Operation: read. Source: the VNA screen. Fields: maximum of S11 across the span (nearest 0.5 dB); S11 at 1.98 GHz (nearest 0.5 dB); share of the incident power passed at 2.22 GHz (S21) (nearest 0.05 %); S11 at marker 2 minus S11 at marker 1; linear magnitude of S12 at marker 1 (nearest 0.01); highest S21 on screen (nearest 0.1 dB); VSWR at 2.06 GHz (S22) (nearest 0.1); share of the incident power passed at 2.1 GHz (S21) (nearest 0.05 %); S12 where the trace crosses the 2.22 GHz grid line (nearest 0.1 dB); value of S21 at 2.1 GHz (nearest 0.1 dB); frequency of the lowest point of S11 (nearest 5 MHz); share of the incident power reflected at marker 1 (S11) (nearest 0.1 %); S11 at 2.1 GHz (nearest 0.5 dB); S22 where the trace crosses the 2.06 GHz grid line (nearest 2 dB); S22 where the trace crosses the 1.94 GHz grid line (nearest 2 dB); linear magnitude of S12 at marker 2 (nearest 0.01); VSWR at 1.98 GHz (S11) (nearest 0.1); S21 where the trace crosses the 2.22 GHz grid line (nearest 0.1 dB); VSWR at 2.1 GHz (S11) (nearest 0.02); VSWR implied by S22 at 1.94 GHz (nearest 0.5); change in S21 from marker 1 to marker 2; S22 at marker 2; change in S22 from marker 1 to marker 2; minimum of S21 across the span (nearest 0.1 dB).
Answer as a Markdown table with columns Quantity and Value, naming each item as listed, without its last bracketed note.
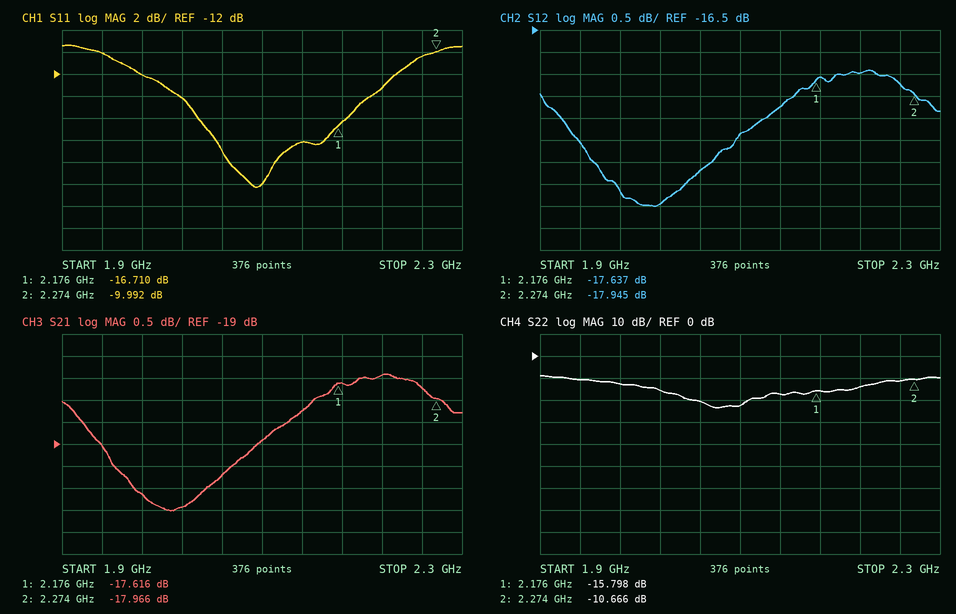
| Quantity | Value |
|---|---|
| maximum of S11 across the span | -9.5 dB |
| S11 at 1.98 GHz | -12.0 dB |
| share of the incident power passed at 2.22 GHz (S21) | 1.80 % |
| S11 at marker 2 minus S11 at marker 1 | 6.718 dB |
| linear magnitude of S12 at marker 1 | 0.13 |
| highest S21 on screen | -17.4 dB |
| VSWR at 2.06 GHz (S22) | 1.2 |
| share of the incident power passed at 2.1 GHz (S21) | 1.30 % |
| S12 where the trace crosses the 2.22 GHz grid line | -17.5 dB |
| value of S21 at 2.1 GHz | -18.9 dB |
| frequency of the lowest point of S11 | 2.095 GHz |
| share of the incident power reflected at marker 1 (S11) | 2.1 % |
| S11 at 2.1 GHz | -22.0 dB |
| S22 where the trace crosses the 2.06 GHz grid line | -20 dB |
| S22 where the trace crosses the 1.94 GHz grid line | -10 dB |
| linear magnitude of S12 at marker 2 | 0.13 |
| VSWR at 1.98 GHz (S11) | 1.7 |
| S21 where the trace crosses the 2.22 GHz grid line | -17.4 dB |
| VSWR at 2.1 GHz (S11) | 1.18 |
| VSWR implied by S22 at 1.94 GHz | 2.0 |
| change in S21 from marker 1 to marker 2 | -0.350 dB |
| S22 at marker 2 | -10.666 dB |
| change in S22 from marker 1 to marker 2 | 5.132 dB |
| minimum of S21 across the span | -20.5 dB |
